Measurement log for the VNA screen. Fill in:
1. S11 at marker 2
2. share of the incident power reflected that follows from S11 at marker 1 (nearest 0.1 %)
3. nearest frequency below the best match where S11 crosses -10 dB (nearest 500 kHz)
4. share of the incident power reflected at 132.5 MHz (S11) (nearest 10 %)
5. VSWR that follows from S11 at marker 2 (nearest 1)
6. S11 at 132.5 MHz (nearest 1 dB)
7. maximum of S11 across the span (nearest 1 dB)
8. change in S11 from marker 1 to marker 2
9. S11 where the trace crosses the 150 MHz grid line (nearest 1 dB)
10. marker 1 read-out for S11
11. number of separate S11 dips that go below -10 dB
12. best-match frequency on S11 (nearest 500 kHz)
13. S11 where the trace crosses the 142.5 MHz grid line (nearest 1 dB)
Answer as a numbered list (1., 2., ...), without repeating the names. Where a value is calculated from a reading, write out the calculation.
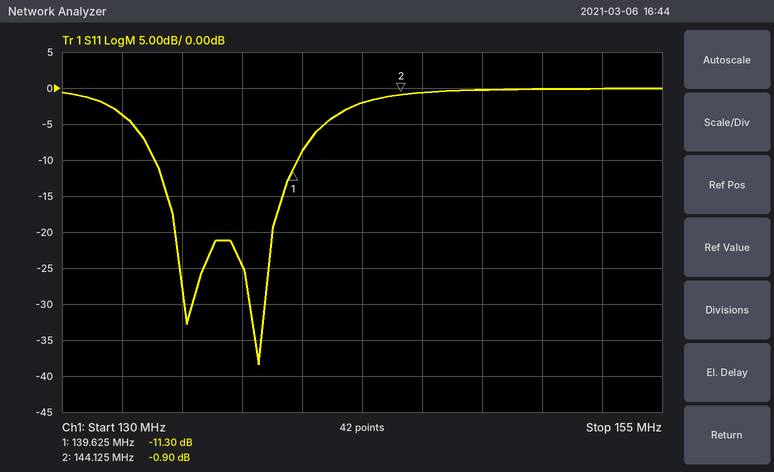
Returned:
1. -0.90 dB
2. 10^(-11.3/10) ≈ 7.4 %
3. 134.0 MHz
4. 10^(-4/10) ≈ 40 %
5. (1 + 0.9016)/(1 − 0.9016) ≈ 19
6. -4 dB
7. 0 dB
8. -0.9 − (-11.3) = 10.40 dB
9. 0 dB
10. -11.30 dB
11. 2
12. 138.0 MHz
13. -2 dB
